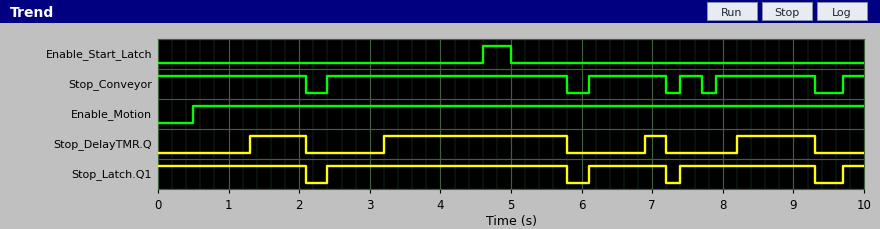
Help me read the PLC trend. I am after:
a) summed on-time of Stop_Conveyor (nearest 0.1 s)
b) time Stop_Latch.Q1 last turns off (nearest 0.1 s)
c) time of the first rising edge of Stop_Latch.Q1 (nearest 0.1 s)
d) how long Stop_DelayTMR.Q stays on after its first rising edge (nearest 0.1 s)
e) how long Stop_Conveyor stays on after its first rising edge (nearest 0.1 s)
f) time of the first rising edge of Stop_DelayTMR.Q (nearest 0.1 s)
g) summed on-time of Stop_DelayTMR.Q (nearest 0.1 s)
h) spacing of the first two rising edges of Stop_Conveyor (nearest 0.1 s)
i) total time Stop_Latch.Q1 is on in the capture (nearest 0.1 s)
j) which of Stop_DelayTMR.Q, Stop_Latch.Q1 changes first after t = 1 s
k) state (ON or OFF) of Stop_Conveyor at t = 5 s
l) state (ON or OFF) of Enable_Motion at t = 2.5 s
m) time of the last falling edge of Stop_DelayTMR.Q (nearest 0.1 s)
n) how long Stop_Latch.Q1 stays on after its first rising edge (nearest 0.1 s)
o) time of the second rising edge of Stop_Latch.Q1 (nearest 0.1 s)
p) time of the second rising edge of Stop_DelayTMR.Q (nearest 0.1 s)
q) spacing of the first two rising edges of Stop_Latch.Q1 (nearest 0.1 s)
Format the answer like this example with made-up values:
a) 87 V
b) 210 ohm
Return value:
a) 8.6 s
b) 9.3 s
c) 2.4 s
d) 0.8 s
e) 3.4 s
f) 1.3 s
g) 4.8 s
h) 3.7 s
i) 8.8 s
j) Stop_DelayTMR.Q
k) ON
l) ON
m) 9.3 s
n) 3.4 s
o) 6.1 s
p) 3.2 s
q) 3.7 s
